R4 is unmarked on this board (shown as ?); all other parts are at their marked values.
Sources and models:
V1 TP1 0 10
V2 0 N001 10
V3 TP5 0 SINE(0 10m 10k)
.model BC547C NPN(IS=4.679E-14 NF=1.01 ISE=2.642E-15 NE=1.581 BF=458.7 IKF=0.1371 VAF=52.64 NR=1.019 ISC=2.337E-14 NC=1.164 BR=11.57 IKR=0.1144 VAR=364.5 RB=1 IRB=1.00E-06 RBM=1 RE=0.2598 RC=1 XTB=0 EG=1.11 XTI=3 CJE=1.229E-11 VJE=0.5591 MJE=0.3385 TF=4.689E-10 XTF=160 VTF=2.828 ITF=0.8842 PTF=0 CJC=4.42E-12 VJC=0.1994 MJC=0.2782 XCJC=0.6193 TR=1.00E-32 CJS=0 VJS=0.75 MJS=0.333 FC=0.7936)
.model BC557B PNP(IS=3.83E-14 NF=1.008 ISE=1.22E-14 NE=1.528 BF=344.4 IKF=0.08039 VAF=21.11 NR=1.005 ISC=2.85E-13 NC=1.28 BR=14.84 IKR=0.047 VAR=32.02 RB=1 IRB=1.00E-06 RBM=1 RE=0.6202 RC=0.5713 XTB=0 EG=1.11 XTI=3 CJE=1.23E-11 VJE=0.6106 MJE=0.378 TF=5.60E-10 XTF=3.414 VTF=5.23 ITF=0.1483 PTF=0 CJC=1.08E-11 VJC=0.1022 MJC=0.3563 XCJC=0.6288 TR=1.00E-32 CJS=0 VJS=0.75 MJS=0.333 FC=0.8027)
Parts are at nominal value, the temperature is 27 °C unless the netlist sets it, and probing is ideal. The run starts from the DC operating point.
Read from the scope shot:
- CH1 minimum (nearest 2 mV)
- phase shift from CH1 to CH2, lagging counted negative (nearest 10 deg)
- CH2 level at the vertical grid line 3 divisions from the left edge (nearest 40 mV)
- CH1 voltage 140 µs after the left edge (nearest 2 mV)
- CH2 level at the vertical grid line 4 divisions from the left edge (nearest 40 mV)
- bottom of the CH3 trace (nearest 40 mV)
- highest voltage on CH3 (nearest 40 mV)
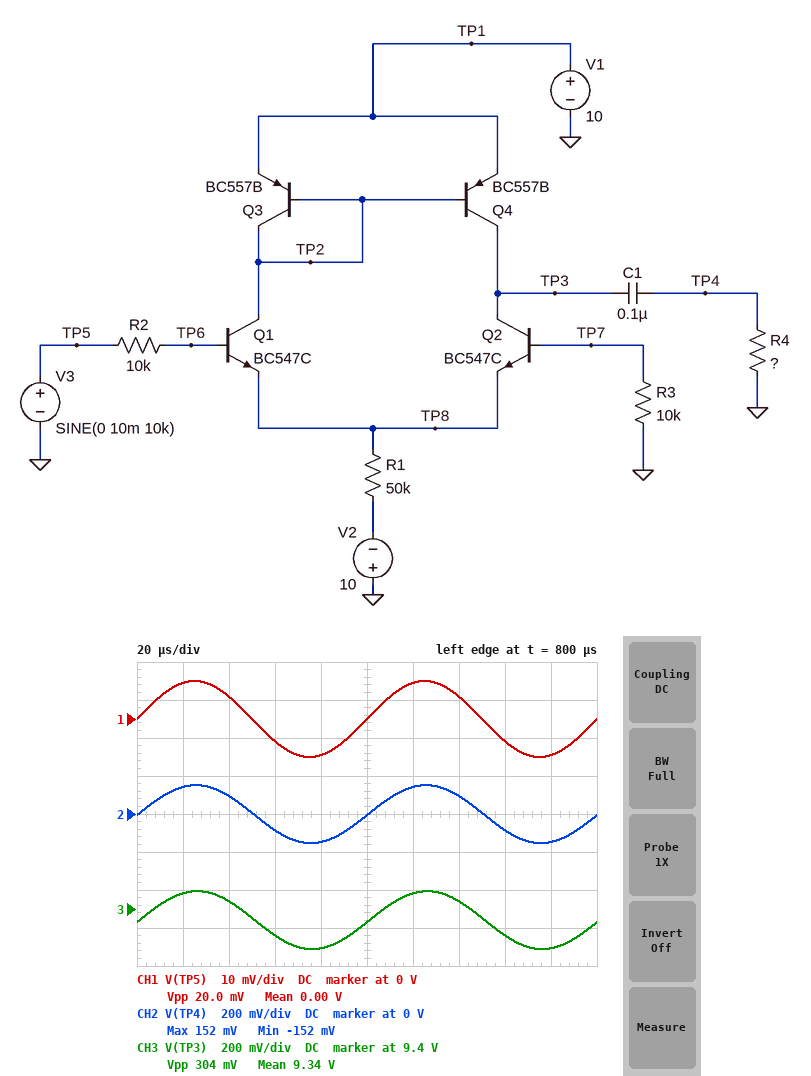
-10 mV
0 deg
-80 mV
6 mV
-160 mV
9.20 V
9.48 V
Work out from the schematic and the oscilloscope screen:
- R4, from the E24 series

4.7 kΩ
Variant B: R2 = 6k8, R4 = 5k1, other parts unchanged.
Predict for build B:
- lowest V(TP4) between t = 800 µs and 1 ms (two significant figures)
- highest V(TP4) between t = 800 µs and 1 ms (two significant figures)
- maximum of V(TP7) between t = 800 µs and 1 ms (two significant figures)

-170 mV
160 mV
-1.3 mV
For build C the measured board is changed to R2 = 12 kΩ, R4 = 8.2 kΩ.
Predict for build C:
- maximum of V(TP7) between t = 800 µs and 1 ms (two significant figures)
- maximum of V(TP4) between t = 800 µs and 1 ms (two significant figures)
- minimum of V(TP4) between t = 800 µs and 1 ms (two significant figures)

-1.3 mV
260 mV
-260 mV
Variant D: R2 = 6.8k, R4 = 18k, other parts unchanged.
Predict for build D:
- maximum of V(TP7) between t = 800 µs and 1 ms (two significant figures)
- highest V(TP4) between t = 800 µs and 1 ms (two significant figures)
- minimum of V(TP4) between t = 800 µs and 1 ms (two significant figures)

-1.1 mV
310 mV
-550 mV
